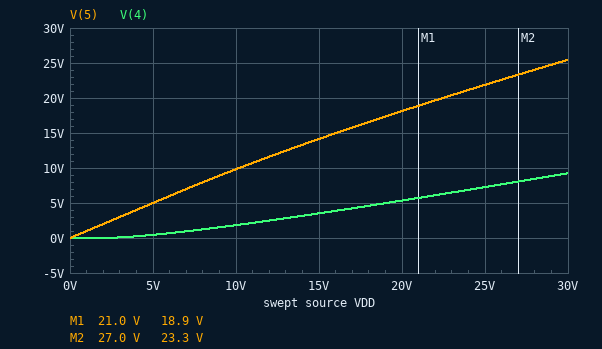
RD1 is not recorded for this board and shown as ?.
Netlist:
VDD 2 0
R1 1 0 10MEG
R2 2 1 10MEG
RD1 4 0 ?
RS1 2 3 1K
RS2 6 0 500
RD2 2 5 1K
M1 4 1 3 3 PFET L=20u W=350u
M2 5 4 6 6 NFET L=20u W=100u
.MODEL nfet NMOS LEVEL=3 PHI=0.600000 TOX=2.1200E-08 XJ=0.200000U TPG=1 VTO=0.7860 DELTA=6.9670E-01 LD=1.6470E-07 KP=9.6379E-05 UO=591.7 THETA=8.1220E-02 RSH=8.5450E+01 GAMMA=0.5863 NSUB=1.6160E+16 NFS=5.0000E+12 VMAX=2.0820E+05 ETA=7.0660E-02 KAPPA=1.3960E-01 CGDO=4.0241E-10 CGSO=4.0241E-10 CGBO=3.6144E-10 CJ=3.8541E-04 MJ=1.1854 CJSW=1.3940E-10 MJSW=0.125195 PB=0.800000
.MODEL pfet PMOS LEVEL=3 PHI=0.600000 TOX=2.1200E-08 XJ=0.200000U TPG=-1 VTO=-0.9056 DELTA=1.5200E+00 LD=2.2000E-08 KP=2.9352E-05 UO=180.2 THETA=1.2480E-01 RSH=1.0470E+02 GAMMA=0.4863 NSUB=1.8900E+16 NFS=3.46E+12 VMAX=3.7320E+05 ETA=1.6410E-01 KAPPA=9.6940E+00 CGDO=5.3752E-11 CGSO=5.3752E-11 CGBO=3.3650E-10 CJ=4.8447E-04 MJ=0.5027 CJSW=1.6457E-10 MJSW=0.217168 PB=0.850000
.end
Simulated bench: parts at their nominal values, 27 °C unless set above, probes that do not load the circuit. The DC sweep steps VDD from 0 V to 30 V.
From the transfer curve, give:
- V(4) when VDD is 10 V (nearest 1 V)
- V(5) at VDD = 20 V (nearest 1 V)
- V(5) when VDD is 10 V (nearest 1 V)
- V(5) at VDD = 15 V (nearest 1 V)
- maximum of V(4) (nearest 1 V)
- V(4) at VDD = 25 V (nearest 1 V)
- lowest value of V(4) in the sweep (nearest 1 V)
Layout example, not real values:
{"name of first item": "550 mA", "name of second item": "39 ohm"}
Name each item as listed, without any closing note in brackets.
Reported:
{"V(4) when VDD is 10 V": "2 V", "V(5) at VDD = 20 V": "18 V", "V(5) when VDD is 10 V": "10 V", "V(5) at VDD = 15 V": "14 V", "maximum of V(4)": "9 V", "V(4) at VDD = 25 V": "7 V", "lowest value of V(4) in the sweep": "0 V"}
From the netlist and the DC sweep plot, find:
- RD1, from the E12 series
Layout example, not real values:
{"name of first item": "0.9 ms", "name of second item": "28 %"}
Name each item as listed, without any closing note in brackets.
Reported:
{"RD1, from the E12 series": "1.5 kΩ"}
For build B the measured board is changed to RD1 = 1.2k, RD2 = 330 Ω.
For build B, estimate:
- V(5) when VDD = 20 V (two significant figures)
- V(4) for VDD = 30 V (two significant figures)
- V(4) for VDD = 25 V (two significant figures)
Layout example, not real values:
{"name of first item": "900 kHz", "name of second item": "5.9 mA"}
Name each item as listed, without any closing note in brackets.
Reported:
{"V(5) when VDD = 20 V": "20 V", "V(4) for VDD = 30 V": "7.4 V", "V(4) for VDD = 25 V": "5.8 V"}
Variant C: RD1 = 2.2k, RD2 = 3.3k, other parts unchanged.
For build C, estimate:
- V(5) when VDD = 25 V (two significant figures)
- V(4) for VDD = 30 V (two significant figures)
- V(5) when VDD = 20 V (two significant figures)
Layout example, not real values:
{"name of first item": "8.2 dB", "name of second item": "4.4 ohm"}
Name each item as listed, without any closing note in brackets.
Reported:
{"V(5) when VDD = 25 V": "7.5 V", "V(4) for VDD = 30 V": "14 V", "V(5) when VDD = 20 V": "8.4 V"}
